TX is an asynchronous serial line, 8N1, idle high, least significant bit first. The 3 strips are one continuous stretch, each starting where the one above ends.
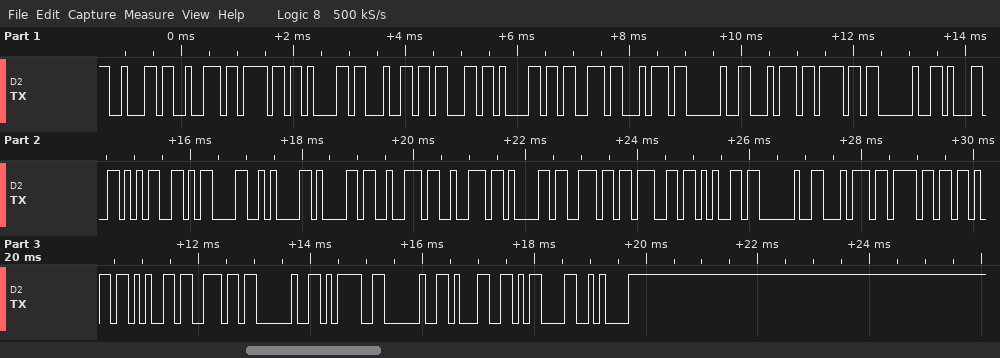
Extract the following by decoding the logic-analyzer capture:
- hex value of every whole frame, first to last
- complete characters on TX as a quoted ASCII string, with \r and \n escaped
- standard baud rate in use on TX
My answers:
62 72 6F 61 64 63 61 73 74 20 74 6F 20 31 35 0D 0A 61 72 72 61 6E 67 65 20 74 6F 6B 65 6E 20 3D 20 31 0D 0A
"broadcast to 15\r\narrange token = 1\r\n"
9600 baud
